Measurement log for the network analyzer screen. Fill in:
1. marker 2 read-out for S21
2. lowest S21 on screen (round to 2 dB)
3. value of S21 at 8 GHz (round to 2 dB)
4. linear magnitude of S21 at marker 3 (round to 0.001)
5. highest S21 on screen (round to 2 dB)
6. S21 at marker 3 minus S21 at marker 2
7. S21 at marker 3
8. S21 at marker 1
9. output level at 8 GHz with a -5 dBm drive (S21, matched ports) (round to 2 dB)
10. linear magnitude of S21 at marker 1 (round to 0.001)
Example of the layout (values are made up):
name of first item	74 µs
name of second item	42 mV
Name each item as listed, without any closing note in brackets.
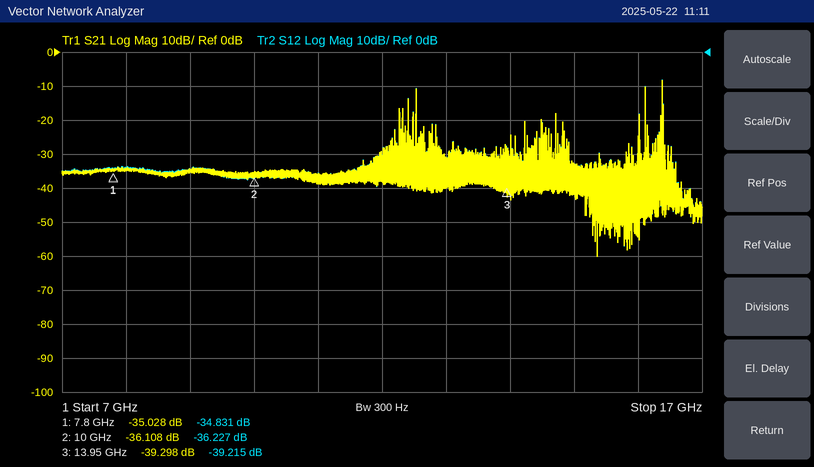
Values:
marker 2 read-out for S21	-36.108 dB
lowest S21 on screen	-60 dB
value of S21 at 8 GHz	-34 dB
linear magnitude of S21 at marker 3	0.011
highest S21 on screen	-8 dB
S21 at marker 3 minus S21 at marker 2	-3.190 dB
S21 at marker 3	-39.298 dB
S21 at marker 1	-35.028 dB
output level at 8 GHz with a -5 dBm drive (S21, matched ports)	-40 dBm
linear magnitude of S21 at marker 1	0.018
